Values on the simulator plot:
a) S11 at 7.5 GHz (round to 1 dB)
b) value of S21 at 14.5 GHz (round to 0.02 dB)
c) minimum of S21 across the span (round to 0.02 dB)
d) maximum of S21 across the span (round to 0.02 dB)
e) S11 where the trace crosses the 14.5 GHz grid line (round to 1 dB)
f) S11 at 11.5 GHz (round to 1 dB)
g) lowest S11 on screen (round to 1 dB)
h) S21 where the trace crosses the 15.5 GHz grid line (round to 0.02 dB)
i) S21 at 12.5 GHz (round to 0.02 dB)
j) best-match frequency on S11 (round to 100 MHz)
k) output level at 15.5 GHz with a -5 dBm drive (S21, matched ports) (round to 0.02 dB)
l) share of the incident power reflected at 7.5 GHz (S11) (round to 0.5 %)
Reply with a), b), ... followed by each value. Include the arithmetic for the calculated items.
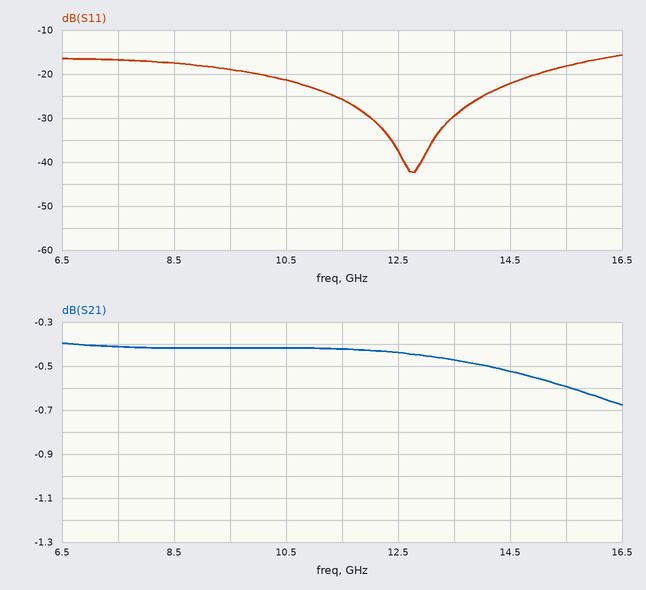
a) -17 dB
b) -0.52 dB
c) -0.68 dB
d) -0.40 dB
e) -22 dB
f) -26 dB
g) -42 dB
h) -0.60 dB
i) -0.44 dB
j) 12.8 GHz
k) -5 dBm + (-0.60 dB) = -5.60 dBm
l) 10^(-17/10) ≈ 2.0 %
